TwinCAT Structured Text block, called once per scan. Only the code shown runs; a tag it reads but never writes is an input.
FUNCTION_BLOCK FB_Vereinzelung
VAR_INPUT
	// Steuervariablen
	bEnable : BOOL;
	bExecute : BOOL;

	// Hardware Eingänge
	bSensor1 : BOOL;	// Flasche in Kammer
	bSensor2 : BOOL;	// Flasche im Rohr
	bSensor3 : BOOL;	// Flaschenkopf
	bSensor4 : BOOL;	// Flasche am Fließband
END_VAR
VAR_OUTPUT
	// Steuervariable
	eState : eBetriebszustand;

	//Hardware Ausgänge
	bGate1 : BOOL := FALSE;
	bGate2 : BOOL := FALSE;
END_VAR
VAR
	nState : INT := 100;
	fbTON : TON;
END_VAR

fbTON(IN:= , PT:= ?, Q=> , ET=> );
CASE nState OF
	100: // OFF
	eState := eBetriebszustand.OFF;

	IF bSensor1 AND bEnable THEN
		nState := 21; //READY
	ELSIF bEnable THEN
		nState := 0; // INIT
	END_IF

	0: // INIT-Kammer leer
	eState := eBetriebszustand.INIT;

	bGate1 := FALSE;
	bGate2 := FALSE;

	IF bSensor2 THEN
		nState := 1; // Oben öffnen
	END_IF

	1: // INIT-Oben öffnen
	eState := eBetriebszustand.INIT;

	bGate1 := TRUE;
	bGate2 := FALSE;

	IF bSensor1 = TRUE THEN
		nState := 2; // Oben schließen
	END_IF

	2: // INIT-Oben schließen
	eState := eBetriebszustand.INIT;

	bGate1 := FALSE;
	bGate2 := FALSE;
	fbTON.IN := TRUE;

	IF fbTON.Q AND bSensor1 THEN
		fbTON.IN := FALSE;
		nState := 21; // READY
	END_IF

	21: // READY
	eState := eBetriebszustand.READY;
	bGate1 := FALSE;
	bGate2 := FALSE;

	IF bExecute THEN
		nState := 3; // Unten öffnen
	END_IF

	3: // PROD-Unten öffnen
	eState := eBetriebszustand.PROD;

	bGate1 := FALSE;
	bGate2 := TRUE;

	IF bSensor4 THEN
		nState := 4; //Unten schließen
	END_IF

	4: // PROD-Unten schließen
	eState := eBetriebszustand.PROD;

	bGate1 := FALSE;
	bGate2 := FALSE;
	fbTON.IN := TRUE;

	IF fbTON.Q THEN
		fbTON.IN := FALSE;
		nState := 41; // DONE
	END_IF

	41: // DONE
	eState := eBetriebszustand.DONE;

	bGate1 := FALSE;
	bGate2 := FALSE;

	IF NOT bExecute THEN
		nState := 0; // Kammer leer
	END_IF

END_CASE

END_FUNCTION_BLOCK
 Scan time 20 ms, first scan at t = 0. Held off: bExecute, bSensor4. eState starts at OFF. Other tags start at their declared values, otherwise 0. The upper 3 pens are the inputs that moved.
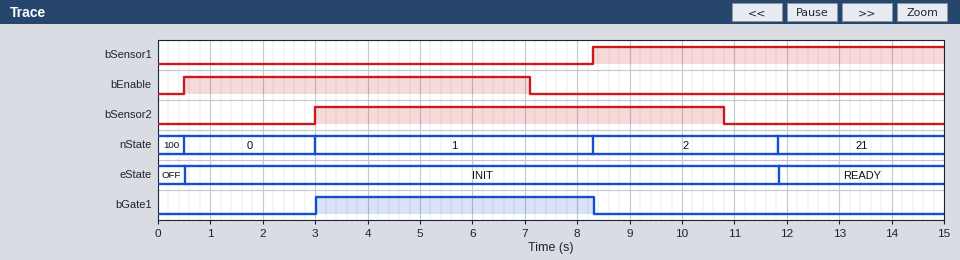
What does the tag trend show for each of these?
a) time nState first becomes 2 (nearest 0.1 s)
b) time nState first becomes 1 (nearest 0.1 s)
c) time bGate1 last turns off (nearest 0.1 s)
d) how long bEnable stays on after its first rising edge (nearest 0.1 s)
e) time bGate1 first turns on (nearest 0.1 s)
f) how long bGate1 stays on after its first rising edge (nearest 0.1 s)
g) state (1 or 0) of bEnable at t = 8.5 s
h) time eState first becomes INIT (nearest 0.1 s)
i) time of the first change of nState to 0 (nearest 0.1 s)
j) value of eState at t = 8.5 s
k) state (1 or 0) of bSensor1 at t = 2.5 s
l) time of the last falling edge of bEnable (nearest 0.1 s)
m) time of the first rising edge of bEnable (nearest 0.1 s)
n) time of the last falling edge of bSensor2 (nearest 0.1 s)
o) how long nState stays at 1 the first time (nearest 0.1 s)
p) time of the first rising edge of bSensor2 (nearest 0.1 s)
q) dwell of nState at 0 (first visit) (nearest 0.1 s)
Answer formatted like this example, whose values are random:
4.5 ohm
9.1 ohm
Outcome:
8.3 s
3.0 s
8.3 s
6.6 s
3.0 s
5.3 s
0
0.5 s
0.5 s
INIT
0
7.1 s
0.5 s
10.8 s
5.3 s
3.0 s
2.5 s
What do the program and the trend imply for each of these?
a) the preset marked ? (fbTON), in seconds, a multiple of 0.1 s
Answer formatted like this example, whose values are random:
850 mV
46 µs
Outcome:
3.5 s
